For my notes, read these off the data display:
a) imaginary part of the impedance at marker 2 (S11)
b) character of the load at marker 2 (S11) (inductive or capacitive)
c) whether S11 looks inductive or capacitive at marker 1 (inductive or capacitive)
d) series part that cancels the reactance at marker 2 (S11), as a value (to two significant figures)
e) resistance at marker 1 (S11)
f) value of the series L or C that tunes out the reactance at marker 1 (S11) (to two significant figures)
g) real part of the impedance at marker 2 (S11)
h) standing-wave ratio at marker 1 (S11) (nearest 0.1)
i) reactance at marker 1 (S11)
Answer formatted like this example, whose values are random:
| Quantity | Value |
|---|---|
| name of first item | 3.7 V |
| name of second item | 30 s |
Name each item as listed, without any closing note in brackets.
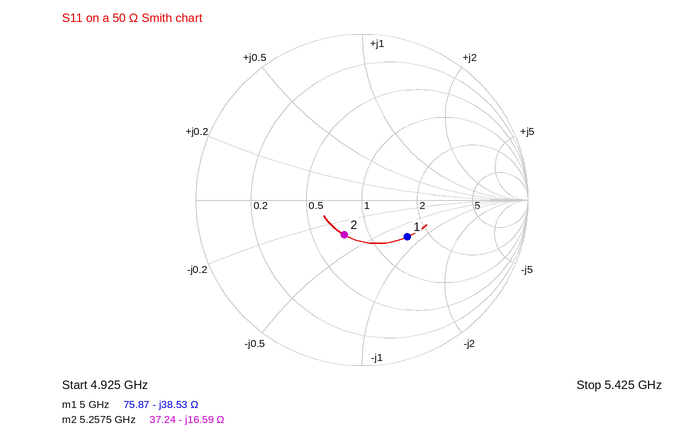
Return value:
| Quantity | Value |
|---|---|
| imaginary part of the impedance at marker 2 | -16.59 Ω |
| character of the load at marker 2 (S11) | capacitive |
| whether S11 looks inductive or capacitive at marker 1 | capacitive |
| series part that cancels the reactance at marker 2 (S11), as a value | 500 pH |
| resistance at marker 1 | 75.87 Ω |
| value of the series L or C that tunes out the reactance at marker 1 (S11) | 1.2 nH |
| real part of the impedance at marker 2 | 37.24 Ω |
| standing-wave ratio at marker 1 (S11) | 2.1 |
| reactance at marker 1 | -38.53 Ω |
